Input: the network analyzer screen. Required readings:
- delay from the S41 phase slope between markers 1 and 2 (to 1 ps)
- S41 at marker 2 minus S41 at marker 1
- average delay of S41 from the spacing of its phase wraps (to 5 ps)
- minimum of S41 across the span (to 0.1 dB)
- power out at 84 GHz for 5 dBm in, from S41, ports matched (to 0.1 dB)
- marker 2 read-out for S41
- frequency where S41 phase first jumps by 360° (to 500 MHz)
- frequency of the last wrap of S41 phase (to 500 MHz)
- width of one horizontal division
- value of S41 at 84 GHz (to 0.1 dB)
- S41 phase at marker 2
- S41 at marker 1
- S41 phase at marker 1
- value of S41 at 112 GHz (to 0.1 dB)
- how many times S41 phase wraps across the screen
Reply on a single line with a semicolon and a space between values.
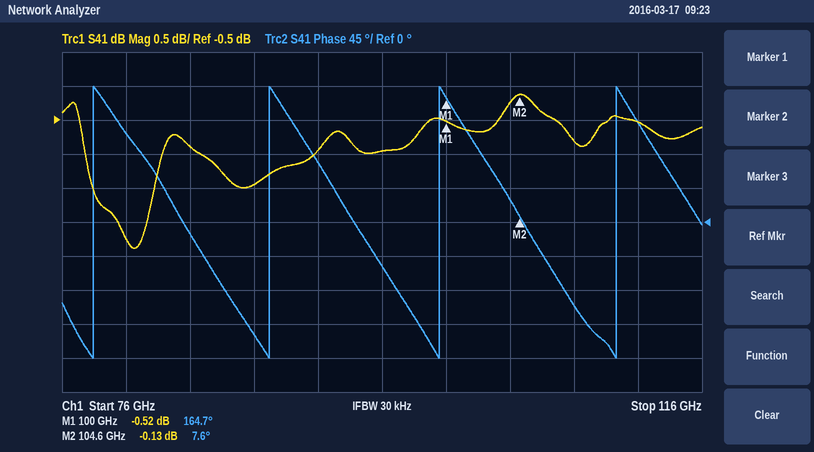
95 ps; 0.39 dB; 90 ps; -2.4 dB; 4.1 dBm; -0.13 dB; 78.0 GHz; 110.5 GHz; 4 GHz; -0.9 dB; 7.6°; -0.52 dB; 164.7°; -0.5 dB; 4
